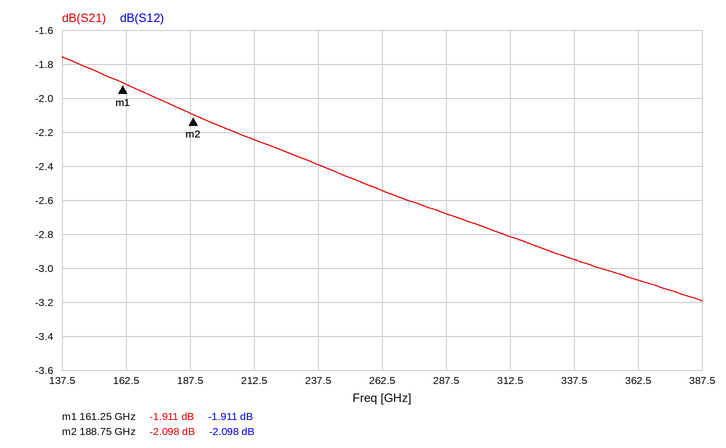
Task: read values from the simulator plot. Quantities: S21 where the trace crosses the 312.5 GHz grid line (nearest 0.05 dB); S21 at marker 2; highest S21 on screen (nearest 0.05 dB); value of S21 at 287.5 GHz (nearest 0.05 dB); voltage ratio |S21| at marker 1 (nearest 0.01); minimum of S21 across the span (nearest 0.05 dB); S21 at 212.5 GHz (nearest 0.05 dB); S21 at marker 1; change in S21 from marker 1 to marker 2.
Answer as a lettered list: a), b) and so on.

a) -2.80 dB
b) -2.098 dB
c) -1.75 dB
d) -2.70 dB
e) 0.80
f) -3.20 dB
g) -2.25 dB
h) -1.911 dB
i) -0.187 dB
